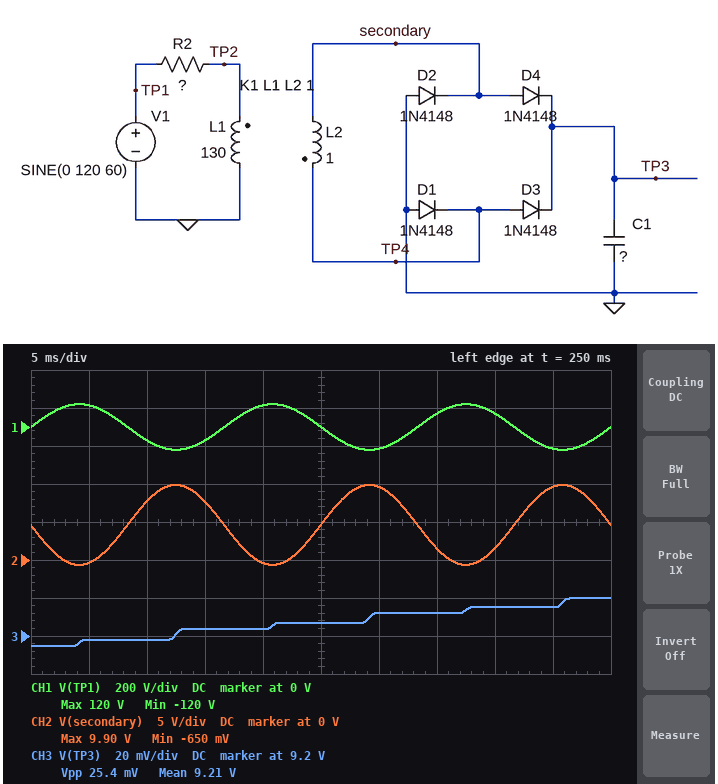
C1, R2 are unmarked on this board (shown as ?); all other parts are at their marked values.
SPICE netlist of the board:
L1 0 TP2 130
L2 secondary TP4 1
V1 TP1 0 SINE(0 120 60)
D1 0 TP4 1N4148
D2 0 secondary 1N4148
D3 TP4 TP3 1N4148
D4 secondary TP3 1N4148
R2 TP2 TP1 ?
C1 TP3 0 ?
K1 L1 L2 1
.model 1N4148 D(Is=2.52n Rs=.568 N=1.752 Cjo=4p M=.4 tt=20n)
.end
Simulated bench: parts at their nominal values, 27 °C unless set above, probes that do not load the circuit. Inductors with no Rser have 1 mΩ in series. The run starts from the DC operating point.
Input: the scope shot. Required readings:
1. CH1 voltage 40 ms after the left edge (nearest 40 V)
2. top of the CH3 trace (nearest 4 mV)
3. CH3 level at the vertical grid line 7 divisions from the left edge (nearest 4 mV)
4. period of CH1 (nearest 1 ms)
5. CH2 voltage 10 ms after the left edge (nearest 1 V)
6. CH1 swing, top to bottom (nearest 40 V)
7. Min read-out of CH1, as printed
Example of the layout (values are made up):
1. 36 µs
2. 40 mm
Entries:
1. 80 V
2. 9.220 V
3. 9.212 V
4. 17 ms
5. 8 V
6. 240 V
7. -120 V
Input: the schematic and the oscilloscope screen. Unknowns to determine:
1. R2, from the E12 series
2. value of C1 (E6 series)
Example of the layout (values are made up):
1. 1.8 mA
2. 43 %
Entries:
1. 330 Ω
2. 680 µF
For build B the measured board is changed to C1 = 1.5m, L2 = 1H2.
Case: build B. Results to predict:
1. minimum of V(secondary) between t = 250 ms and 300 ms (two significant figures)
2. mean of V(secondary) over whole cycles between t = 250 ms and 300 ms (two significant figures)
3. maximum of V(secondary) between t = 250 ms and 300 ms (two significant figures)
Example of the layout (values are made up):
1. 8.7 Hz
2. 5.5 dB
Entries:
1. -720 mV
2. 5.0 V
3. 11 V
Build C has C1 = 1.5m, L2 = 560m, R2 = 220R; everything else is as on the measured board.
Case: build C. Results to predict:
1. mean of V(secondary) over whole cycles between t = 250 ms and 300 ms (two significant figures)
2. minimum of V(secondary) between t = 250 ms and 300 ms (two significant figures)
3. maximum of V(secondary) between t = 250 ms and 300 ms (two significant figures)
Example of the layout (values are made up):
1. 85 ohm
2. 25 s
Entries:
1. 3.3 V
2. -680 mV
3. 7.2 V
